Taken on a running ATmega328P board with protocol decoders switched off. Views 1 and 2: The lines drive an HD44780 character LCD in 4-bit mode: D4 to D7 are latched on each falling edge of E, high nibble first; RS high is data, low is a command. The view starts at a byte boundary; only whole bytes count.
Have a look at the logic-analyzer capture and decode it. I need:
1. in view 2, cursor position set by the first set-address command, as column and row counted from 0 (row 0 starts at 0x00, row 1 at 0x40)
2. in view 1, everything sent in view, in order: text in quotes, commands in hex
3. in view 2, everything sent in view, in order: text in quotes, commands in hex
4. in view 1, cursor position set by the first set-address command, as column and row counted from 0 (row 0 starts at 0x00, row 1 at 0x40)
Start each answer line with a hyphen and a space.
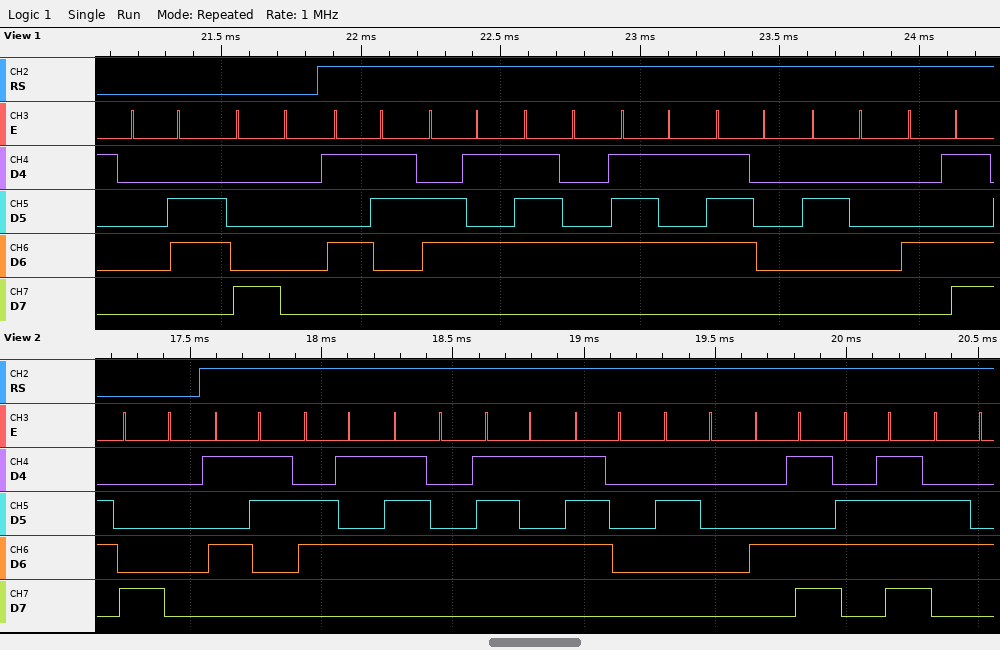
- column 0, row 0
- 0x06 0x80 "Setup M"
- 0x80 "Setup Mod"
- column 0, row 0
